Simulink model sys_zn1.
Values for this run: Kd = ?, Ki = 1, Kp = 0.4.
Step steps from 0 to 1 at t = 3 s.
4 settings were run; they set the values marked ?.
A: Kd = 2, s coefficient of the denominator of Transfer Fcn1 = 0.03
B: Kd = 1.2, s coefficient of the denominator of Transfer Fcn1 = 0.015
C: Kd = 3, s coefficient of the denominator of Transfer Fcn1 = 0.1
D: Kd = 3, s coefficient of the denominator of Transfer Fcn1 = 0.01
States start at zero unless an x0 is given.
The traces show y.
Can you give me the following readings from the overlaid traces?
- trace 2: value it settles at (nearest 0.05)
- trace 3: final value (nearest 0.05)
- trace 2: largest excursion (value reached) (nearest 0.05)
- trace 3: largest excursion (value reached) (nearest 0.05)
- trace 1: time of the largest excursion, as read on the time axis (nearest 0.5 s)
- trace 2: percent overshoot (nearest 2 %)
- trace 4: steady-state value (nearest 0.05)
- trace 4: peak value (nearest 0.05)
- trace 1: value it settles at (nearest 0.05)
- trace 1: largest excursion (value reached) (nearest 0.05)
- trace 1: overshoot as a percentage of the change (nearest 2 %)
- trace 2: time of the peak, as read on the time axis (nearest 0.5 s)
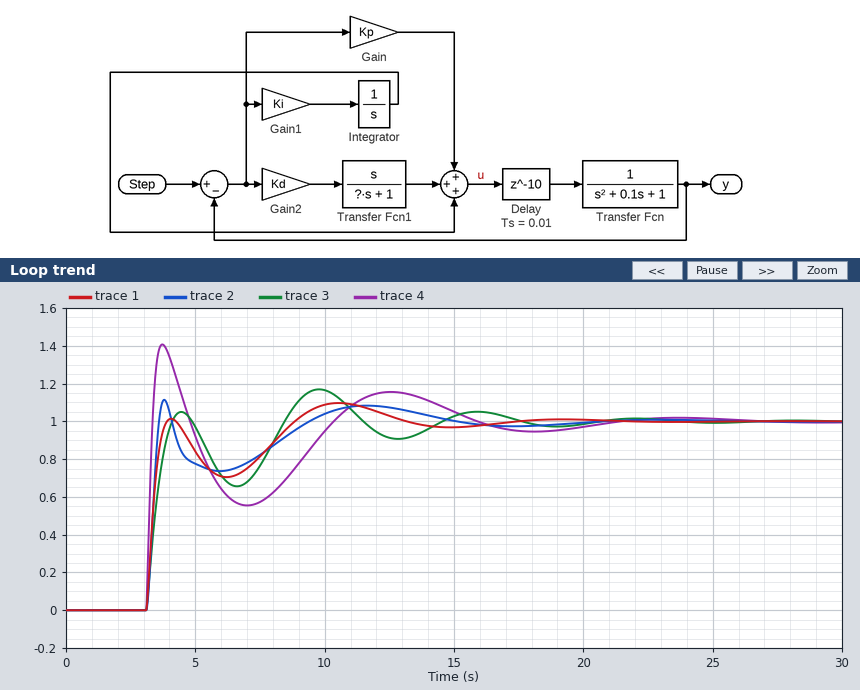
1.00
1.00
1.10
1.15
10.5 s
12 %
1.00
1.40
1.00
1.10
10 %
4.0 s
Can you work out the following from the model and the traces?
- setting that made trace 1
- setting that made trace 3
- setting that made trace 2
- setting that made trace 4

A
B
C
D
